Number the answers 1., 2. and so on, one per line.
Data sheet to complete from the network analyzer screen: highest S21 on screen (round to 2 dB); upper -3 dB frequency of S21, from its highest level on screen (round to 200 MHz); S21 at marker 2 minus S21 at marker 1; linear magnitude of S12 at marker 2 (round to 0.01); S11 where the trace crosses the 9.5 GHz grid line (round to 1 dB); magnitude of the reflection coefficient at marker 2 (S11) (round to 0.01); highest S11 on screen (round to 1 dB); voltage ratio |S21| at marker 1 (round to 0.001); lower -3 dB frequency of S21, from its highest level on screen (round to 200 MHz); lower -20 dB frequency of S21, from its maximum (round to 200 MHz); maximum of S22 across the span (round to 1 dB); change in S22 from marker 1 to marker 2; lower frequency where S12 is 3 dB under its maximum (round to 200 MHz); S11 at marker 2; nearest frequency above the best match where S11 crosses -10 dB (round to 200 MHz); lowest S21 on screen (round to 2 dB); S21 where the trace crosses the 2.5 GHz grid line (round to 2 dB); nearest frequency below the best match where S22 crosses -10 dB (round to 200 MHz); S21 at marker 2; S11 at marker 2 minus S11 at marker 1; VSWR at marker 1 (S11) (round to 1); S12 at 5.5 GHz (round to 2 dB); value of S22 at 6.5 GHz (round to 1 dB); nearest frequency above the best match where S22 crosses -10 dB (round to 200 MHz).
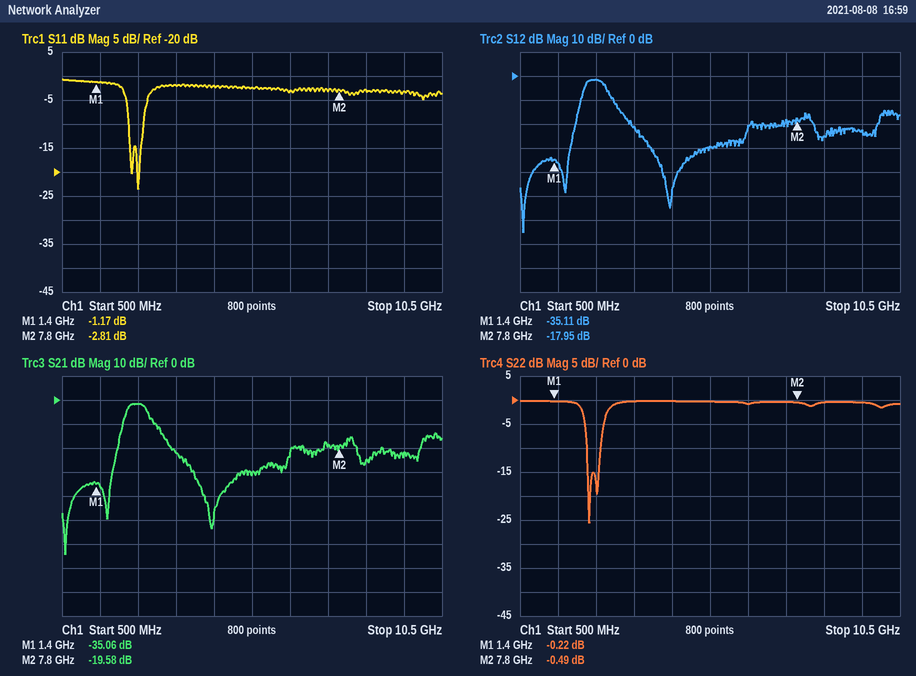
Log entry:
1. -2 dB
2. 2.8 GHz
3. 15.48 dB
4. 0.13
5. -3 dB
6. 0.72
7. -1 dB
8. 0.018
9. 2.2 GHz
10. 2.0 GHz
11. 0 dB
12. -0.27 dB
13. 2.2 GHz
14. -2.81 dB
15. 2.6 GHz
16. -64 dB
17. -2 dB
18. 2.2 GHz
19. -19.58 dB
20. -1.64 dB
21. 15
22. -30 dB
23. -1 dB
24. 2.6 GHz
